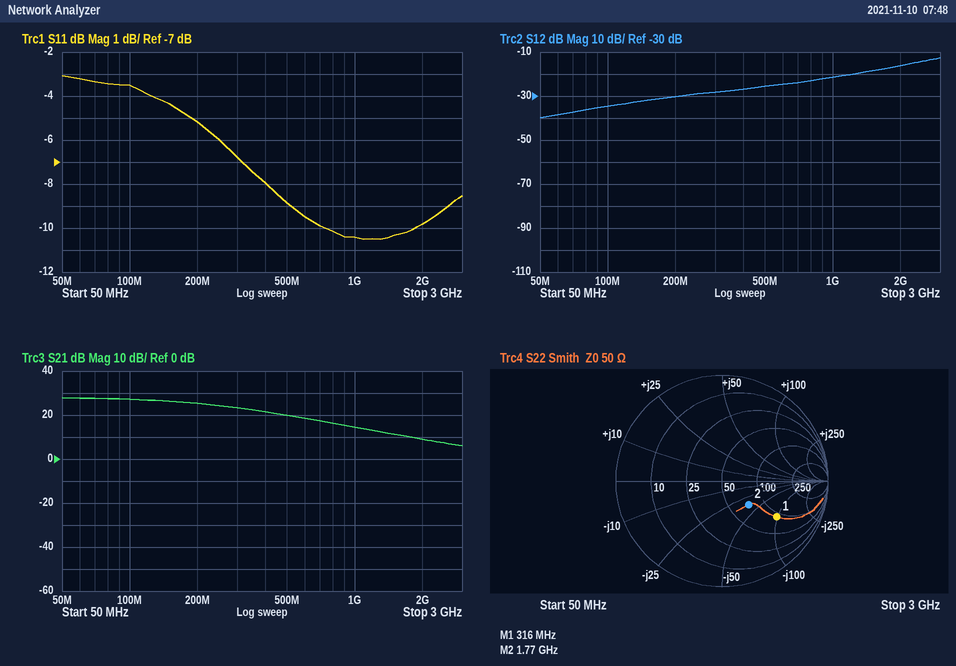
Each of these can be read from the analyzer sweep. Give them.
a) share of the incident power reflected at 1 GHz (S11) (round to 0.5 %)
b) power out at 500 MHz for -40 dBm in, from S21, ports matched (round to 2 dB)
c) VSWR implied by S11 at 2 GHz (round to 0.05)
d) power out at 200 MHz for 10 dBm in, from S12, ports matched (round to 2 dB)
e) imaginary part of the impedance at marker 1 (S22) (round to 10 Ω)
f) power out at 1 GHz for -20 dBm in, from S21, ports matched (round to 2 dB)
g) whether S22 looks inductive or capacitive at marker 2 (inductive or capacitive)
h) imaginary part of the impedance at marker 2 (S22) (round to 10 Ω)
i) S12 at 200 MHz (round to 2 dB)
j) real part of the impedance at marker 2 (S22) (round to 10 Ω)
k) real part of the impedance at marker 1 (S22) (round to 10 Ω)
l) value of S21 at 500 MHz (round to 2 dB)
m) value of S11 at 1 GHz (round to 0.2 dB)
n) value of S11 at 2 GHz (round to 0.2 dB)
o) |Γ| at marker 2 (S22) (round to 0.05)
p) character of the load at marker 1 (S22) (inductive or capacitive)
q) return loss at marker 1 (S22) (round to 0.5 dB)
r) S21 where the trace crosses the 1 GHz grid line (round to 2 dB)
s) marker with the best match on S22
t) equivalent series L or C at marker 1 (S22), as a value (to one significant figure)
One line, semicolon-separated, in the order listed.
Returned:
9.0 %; -20 dBm; 1.95; -20 dBm; -100 Ω; -6 dBm; capacitive; -40 Ω; -30 dB; 70 Ω; 90 Ω; 20 dB; -10.4 dB; -9.8 dB; 0.35; capacitive; 4.0 dB; 14 dB; marker 2; 5 pF
